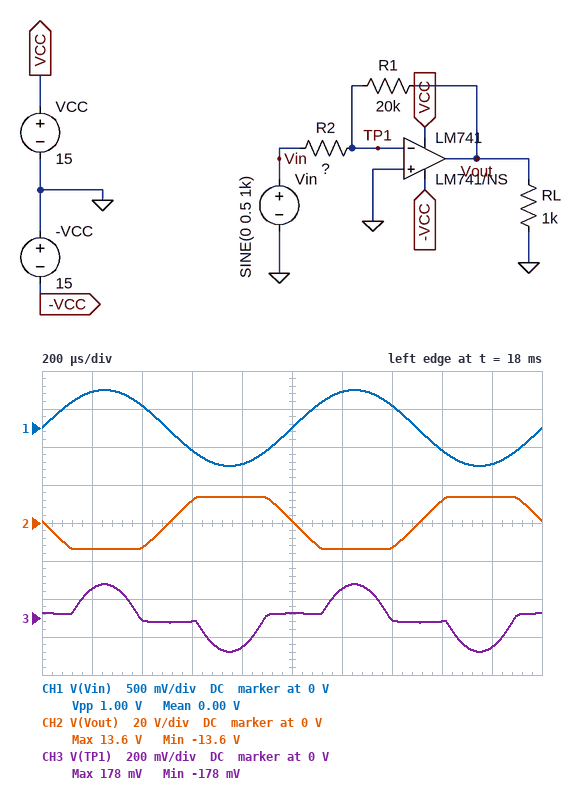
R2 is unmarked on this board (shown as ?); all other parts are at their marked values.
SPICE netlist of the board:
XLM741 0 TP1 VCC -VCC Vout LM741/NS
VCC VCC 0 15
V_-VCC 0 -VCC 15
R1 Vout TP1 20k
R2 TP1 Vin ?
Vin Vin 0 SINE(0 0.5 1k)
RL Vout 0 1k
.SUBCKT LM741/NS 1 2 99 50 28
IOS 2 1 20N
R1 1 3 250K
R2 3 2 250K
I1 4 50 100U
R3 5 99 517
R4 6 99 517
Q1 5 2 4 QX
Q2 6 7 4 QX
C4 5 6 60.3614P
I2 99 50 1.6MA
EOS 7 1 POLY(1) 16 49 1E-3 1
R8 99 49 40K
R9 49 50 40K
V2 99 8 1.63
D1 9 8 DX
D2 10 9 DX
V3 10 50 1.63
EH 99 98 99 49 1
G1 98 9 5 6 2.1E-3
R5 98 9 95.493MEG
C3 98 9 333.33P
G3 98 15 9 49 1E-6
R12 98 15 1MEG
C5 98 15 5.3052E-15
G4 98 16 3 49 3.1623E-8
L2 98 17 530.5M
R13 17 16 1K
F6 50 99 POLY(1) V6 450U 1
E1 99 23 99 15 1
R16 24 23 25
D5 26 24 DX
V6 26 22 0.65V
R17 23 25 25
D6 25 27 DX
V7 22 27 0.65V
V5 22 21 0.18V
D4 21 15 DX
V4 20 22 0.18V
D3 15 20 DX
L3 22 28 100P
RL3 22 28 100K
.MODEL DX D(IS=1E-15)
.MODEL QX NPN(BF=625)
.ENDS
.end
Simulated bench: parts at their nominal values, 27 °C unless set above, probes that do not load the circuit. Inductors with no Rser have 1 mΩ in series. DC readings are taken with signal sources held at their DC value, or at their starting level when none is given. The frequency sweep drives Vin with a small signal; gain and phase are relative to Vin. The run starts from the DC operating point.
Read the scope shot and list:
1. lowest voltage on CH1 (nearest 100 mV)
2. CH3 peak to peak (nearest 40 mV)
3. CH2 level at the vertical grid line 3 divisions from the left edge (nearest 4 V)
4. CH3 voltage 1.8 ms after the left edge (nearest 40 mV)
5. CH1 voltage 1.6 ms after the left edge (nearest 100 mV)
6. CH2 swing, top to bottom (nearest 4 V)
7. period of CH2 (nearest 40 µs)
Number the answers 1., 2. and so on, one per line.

1. -500 mV
2. 360 mV
3. 12 V
4. -160 mV
5. -300 mV
6. 28 V
7. 1.00 ms
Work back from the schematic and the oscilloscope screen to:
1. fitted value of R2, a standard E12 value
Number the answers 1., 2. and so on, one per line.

1. 470 Ω
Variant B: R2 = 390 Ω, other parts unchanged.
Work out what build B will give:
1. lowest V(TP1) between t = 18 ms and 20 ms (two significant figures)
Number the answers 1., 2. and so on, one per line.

1. -230 mV
